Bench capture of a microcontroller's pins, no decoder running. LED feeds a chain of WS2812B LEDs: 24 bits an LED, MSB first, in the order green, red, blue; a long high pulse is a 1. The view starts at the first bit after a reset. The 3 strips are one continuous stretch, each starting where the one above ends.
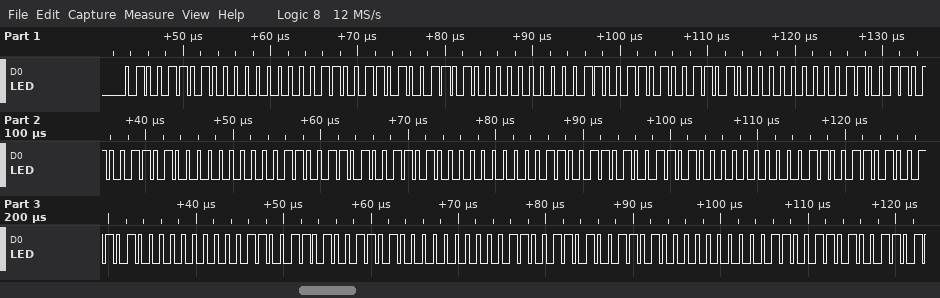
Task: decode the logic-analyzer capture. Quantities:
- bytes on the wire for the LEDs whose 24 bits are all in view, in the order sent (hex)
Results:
4D 00 33 4D 00 33 4D 00 33 4D 00 33 4D 00 33 4D 00 33 4D 00 33 4D 00 33 4D 00 33
